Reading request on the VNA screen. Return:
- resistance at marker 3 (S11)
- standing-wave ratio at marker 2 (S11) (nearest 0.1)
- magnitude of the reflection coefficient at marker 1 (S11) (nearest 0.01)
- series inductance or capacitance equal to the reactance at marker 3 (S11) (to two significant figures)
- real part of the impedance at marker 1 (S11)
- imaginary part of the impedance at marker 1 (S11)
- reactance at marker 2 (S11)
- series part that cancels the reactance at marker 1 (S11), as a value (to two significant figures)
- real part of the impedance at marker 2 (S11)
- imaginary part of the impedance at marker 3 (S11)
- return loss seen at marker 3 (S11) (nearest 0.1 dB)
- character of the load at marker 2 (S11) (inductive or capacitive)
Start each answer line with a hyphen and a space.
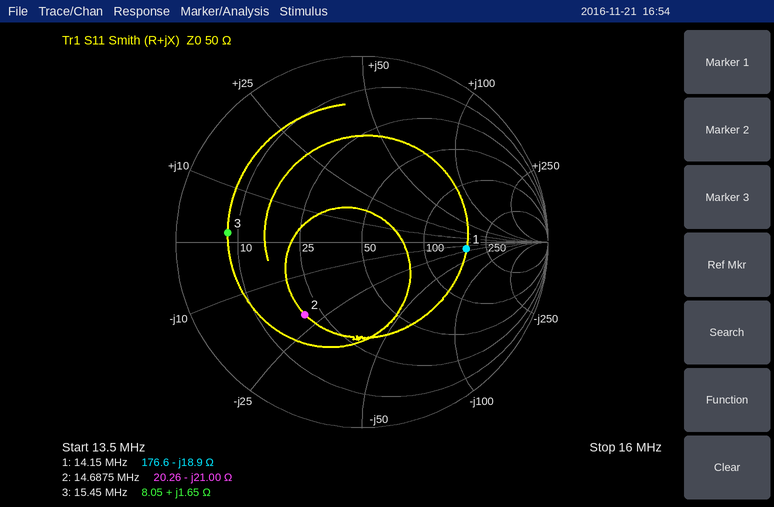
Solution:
- 8.05 Ω
- 3.0
- 0.56
- 17 nH
- 176.6 Ω
- -18.9 Ω
- -21.00 Ω
- 210 nH
- 20.26 Ω
- +1.65 Ω
- 2.8 dB
- capacitive
